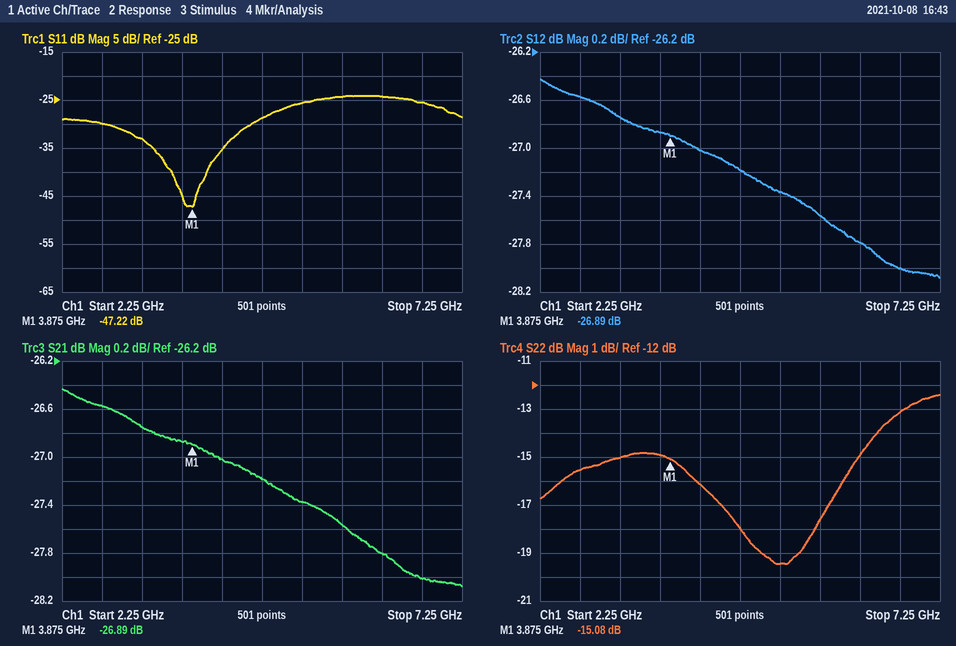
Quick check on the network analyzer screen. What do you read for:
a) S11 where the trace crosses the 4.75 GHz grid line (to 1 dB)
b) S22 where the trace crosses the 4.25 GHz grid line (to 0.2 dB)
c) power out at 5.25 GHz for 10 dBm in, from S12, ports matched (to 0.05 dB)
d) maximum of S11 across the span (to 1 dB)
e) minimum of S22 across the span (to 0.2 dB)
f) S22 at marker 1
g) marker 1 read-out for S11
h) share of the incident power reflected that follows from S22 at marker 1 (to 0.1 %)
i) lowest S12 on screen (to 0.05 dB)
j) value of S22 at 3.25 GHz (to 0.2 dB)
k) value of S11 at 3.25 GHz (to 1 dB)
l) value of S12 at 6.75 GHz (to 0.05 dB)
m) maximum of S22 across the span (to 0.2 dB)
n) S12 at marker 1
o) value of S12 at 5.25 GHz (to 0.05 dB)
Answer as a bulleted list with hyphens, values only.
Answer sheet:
- -29 dB
- -16.2 dB
- -17.35 dBm
- -24 dB
- -19.4 dB
- -15.08 dB
- -47.22 dB
- 3.1 %
- -28.10 dB
- -15.0 dB
- -33 dB
- -28.00 dB
- -12.4 dB
- -26.89 dB
- -27.35 dB
